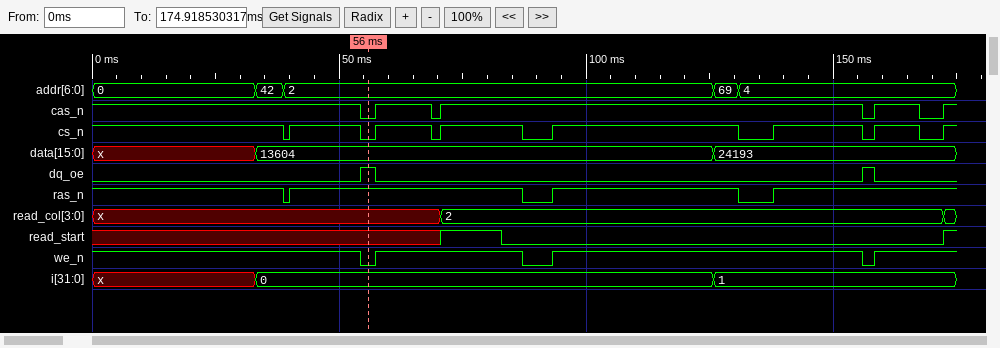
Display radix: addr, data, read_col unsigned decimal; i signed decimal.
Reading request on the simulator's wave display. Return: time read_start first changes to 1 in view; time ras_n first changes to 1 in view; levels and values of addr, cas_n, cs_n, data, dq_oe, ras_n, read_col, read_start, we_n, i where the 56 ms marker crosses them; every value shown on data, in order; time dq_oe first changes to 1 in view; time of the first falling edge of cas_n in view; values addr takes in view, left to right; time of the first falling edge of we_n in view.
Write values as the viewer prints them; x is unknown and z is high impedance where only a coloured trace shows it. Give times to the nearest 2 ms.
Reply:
70 ms
40 ms
addr=2, cas_n=0, cs_n=0, data=13604, dq_oe=1, ras_n=1, read_col=x, read_start=x, we_n=0, i=0
x, 13604, 24193
54 ms
54 ms
0, 42, 2, 69, 4
54 ms
